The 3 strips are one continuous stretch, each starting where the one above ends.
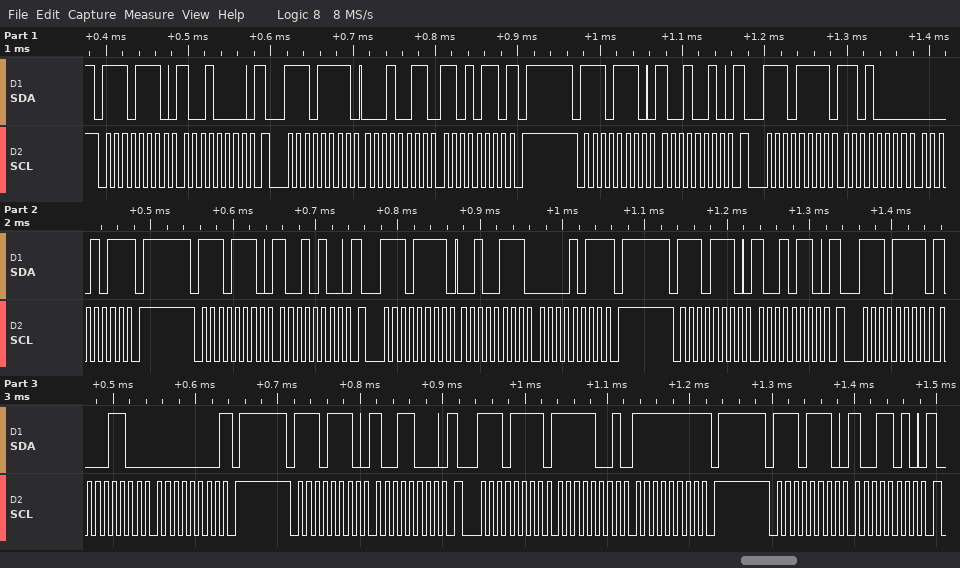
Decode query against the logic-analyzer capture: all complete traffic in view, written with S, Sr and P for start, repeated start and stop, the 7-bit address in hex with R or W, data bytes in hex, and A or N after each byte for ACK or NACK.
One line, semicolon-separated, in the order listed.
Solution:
S 77W A 90 A Sr 77R A 13 A D6 N P S 77W A 92 A Sr 77R A D0 A 0B N P S 77W A 94 A Sr 77R A 27 A 0B N P S 77W A 96 A Sr 77R A 8C A 00 N P S 77W A 98 A Sr 77R A F9 A FF N P S 77W A 9A A
